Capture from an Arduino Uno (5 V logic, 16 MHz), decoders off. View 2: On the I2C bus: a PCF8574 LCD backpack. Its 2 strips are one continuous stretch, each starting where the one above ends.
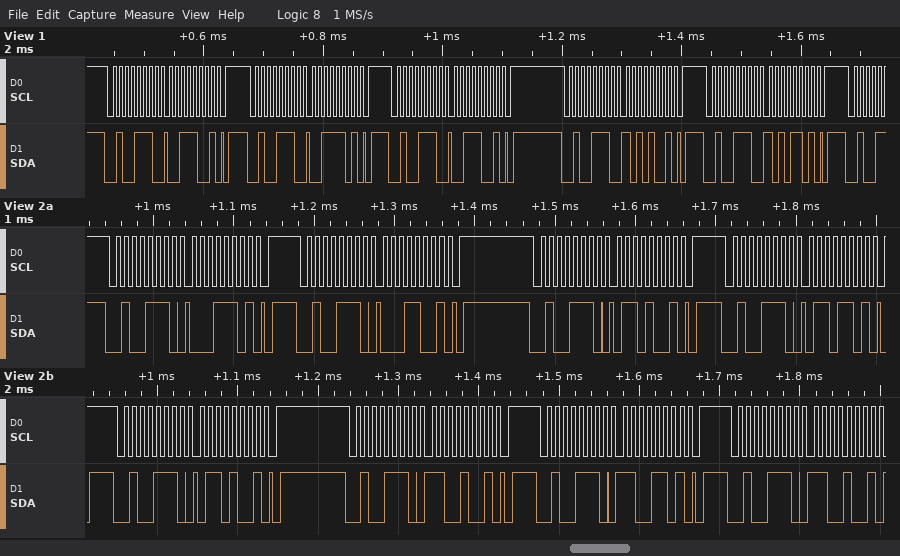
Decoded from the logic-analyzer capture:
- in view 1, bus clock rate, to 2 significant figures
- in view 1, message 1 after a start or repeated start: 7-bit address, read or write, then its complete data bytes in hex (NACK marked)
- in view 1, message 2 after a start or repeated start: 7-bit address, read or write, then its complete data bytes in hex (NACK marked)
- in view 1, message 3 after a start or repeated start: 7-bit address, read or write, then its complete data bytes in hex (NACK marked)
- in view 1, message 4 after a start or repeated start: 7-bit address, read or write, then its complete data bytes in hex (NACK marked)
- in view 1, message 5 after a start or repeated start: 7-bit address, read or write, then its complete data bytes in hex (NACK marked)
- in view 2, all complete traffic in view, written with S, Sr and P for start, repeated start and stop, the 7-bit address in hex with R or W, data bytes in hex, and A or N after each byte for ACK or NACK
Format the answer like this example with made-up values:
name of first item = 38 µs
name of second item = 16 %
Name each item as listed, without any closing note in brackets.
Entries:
in view 1, bus clock rate, to 2 significant figures = 100 kHz
in view 1, message 1 after a start or repeated start: 7-bit address, read or write, then its complete data bytes in hex = 0x27 write: 39
in view 1, message 2 after a start or repeated start: 7-bit address, read or write, then its complete data bytes in hex = 0x27 write: 3D
in view 1, message 3 after a start or repeated start: 7-bit address, read or write, then its complete data bytes in hex = 0x27 write: 39
in view 1, message 4 after a start or repeated start: 7-bit address, read or write, then its complete data bytes in hex = 0x27 write: A9
in view 1, message 5 after a start or repeated start: 7-bit address, read or write, then its complete data bytes in hex = 0x27 write: AD
in view 2, all complete traffic in view, written with S, Sr and P for start, repeated start and stop, the 7-bit address in hex with R or W, data bytes in hex, and A or N after each byte for ACK or NACK = S 27W A 1D A P S 27W A 19 A P S 27W A 69 A P S 27W A 6D A P S 27W A 69 A P S 27W A C9 A P S 27W A CD A P S 27W A C9 A
